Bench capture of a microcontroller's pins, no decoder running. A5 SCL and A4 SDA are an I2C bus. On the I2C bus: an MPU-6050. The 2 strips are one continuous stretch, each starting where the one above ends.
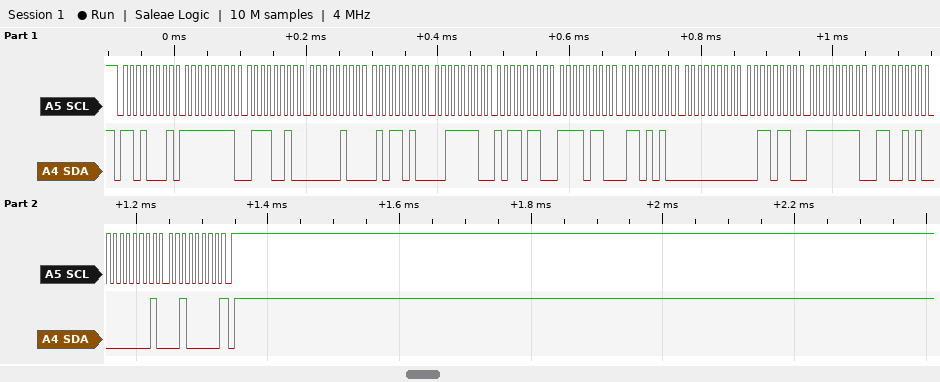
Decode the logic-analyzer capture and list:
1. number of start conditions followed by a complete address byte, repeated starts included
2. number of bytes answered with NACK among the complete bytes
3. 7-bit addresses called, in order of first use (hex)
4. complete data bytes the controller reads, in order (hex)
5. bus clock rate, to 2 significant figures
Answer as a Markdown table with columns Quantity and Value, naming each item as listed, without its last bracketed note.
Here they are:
| Quantity | Value |
|---|---|
| number of start conditions followed by a complete address byte, repeated starts included | 1 |
| number of bytes answered with NACK among the complete bytes | 1 |
| 7-bit addresses called, in order of first use | 0x68 |
| complete data bytes the controller reads, in order | FF 72 04 5A 3E B6 F6 6A 00 36 FF 65 01 20 |
| bus clock rate, to 2 significant figures | 100 kHz |
